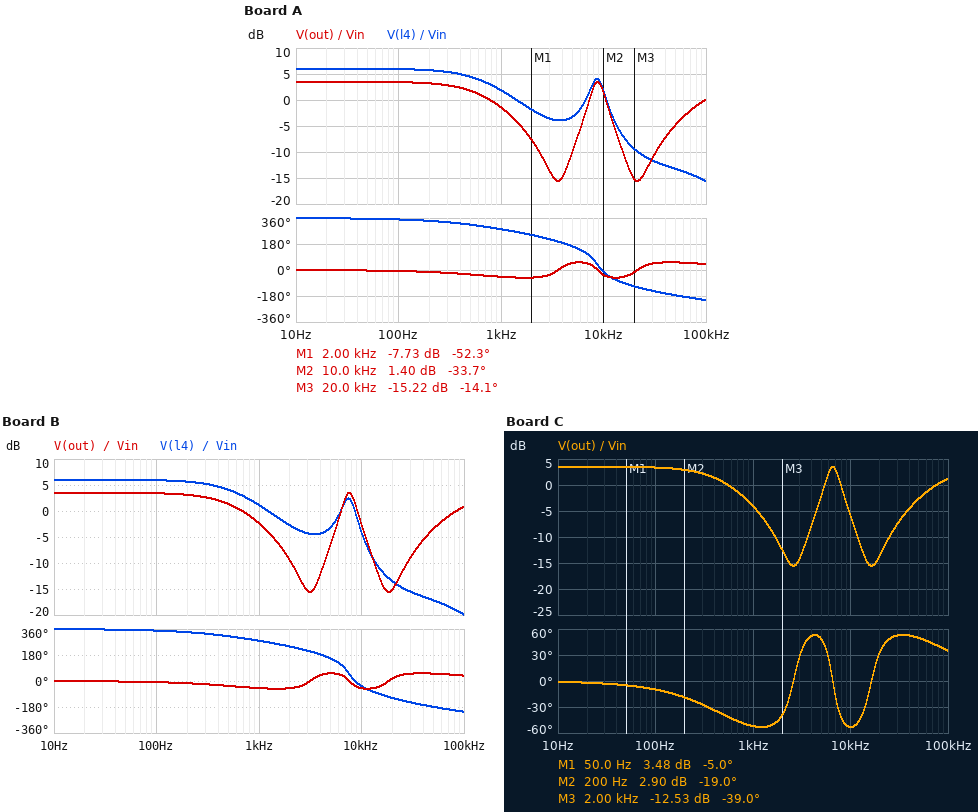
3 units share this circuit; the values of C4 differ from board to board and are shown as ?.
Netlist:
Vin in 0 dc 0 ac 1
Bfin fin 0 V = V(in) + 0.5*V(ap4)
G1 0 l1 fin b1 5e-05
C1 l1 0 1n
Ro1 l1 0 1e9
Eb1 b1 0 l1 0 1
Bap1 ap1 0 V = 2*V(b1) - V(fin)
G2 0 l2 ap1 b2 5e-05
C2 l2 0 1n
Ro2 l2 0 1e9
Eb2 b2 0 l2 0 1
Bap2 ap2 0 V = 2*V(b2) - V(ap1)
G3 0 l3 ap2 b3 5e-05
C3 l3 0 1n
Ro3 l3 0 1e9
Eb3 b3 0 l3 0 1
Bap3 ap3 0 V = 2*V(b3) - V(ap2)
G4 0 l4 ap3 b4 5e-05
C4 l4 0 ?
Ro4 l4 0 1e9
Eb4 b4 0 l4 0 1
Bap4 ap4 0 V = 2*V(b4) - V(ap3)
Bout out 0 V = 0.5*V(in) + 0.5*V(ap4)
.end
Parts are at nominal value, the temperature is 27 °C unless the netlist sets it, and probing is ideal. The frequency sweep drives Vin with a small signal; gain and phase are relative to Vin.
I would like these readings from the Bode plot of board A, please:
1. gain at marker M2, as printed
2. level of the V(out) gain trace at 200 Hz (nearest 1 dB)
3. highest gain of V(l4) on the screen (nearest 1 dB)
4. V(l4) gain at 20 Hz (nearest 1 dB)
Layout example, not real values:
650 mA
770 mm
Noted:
1.40 dB
3 dB
6 dB
6 dB
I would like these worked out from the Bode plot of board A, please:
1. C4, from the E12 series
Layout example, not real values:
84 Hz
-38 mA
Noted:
680 pF
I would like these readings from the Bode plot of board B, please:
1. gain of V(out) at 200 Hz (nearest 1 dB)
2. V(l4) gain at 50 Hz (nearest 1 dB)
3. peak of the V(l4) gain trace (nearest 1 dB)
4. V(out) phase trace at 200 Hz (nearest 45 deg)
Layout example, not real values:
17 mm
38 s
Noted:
3 dB
6 dB
6 dB
0 deg
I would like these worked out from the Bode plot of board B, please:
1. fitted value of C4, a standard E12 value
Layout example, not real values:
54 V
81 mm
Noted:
1.2 nF
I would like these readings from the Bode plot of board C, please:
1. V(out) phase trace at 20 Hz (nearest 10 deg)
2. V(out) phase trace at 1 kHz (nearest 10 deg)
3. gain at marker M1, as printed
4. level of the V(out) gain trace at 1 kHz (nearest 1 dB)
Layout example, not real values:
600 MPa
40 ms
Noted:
0 deg
-50 deg
3.48 dB
-4 dB
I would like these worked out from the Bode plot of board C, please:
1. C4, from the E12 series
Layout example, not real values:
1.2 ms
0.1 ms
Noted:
2.2 nF
